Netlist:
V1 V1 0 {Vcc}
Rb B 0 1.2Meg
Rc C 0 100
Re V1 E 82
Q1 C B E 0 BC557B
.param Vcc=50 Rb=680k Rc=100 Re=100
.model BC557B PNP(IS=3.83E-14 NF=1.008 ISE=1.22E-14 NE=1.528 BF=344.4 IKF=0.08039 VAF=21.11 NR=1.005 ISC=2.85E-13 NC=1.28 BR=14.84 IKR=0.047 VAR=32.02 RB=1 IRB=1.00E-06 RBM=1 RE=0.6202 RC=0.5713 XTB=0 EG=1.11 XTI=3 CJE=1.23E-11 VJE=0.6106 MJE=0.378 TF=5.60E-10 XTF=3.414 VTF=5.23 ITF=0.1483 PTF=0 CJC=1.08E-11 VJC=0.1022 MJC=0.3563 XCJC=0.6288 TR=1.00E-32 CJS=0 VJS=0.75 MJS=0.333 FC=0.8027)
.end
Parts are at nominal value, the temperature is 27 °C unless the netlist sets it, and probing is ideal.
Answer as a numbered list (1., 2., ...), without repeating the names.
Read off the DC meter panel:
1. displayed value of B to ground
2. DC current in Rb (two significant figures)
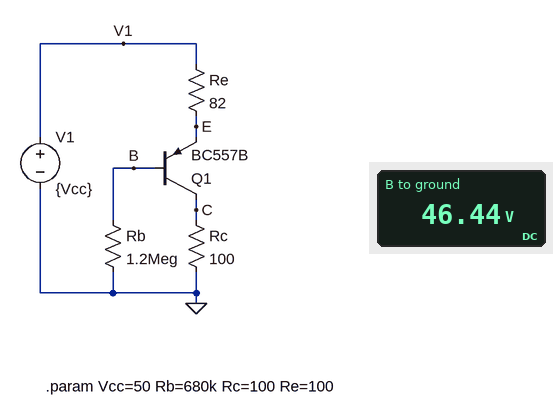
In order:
1. 46.44 V
2. 39 µA
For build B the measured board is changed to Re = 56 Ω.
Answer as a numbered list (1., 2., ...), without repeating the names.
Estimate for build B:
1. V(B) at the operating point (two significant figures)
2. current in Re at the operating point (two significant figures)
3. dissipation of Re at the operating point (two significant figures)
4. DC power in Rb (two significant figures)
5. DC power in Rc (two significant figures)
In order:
1. 47 V
2. 36 mA
3. 71 mW
4. 1.9 mW
5. 130 mW
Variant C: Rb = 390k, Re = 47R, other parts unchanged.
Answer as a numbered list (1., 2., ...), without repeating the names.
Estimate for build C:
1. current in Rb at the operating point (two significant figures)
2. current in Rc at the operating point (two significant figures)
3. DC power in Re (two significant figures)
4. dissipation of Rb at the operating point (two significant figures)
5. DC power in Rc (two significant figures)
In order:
1. 120 µA
2. 80 mA
3. 300 mW
4. 5.3 mW
5. 640 mW
